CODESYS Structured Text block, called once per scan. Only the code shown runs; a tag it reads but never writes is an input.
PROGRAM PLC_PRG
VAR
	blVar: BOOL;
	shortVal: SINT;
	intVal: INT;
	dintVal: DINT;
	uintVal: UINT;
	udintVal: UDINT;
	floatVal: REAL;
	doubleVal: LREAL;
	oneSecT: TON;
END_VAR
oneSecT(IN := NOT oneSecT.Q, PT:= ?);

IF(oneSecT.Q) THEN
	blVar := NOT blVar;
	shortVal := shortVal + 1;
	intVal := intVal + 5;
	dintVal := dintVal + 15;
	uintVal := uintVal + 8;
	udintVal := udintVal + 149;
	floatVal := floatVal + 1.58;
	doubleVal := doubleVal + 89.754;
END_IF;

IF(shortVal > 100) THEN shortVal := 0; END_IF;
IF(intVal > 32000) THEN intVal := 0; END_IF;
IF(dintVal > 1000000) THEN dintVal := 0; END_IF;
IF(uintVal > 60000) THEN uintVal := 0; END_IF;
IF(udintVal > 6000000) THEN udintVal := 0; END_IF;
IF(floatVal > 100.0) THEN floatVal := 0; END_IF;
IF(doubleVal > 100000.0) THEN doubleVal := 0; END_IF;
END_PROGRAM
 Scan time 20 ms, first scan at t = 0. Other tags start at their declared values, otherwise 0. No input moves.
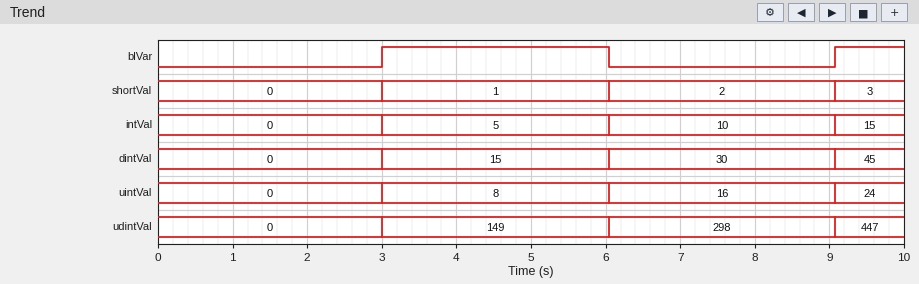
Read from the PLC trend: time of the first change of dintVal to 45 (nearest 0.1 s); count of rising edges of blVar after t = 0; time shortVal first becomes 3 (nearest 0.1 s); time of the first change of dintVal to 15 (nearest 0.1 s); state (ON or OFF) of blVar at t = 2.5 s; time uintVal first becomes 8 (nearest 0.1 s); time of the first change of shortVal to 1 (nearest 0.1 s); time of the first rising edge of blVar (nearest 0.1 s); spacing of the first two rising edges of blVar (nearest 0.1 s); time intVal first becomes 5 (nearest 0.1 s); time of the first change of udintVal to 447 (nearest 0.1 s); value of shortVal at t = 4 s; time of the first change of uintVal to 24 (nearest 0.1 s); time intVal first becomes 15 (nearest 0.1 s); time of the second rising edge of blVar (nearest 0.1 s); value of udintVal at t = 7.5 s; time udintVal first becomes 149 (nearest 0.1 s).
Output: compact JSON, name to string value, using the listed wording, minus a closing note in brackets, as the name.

{"time of the first change of dintVal to 45": "9.1 s", "count of rising edges of blVar after t = 0": "2", "time shortVal first becomes 3": "9.1 s", "time of the first change of dintVal to 15": "3.0 s", "state (ON or OFF) of blVar at t = 2.5 s": "OFF", "time uintVal first becomes 8": "3.0 s", "time of the first change of shortVal to 1": "3.0 s", "time of the first rising edge of blVar": "3.0 s", "spacing of the first two rising edges of blVar": "6.1 s", "time intVal first becomes 5": "3.0 s", "time of the first change of udintVal to 447": "9.1 s", "value of shortVal at t = 4 s": "1", "time of the first change of uintVal to 24": "9.1 s", "time intVal first becomes 15": "9.1 s", "time of the second rising edge of blVar": "9.1 s", "value of udintVal at t = 7.5 s": "298", "time udintVal first becomes 149": "3.0 s"}
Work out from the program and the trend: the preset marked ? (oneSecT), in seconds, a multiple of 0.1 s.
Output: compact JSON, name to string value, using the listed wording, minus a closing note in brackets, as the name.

{"the preset marked ? (oneSecT), in seconds, a multiple of 0.1 s": "3.0 s"}
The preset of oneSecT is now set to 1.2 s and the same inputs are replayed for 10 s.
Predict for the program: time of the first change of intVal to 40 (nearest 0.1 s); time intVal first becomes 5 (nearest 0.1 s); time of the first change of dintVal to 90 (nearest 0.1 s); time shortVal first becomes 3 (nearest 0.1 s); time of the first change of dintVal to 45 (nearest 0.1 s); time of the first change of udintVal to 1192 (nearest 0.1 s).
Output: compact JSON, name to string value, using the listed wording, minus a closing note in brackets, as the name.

{"time of the first change of intVal to 40": "9.9 s", "time intVal first becomes 5": "1.2 s", "time of the first change of dintVal to 90": "7.4 s", "time shortVal first becomes 3": "3.7 s", "time of the first change of dintVal to 45": "3.7 s", "time of the first change of udintVal to 1192": "9.9 s"}
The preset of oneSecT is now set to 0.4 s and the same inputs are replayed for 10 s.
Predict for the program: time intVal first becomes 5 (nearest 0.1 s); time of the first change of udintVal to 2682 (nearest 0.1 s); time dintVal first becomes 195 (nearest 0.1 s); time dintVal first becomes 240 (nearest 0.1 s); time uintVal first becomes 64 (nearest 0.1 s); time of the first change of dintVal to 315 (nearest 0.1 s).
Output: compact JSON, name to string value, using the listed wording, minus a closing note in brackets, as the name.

{"time intVal first becomes 5": "0.4 s", "time of the first change of udintVal to 2682": "7.9 s", "time dintVal first becomes 195": "5.7 s", "time dintVal first becomes 240": "7.0 s", "time uintVal first becomes 64": "3.5 s", "time of the first change of dintVal to 315": "9.2 s"}
